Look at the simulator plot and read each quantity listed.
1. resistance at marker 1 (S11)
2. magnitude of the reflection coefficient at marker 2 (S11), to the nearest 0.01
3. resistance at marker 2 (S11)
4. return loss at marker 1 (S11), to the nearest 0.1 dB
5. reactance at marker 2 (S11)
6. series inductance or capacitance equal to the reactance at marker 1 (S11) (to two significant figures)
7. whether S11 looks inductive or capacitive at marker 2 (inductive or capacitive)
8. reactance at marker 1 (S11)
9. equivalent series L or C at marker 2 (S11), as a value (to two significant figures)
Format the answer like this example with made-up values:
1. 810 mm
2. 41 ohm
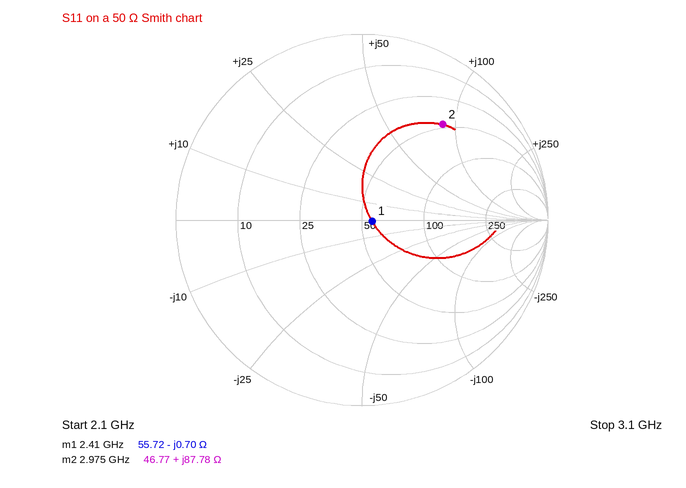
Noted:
1. 55.72 Ω
2. 0.67
3. 46.77 Ω
4. 25.3 dB
5. +87.78 Ω
6. 94 pF
7. inductive
8. -0.70 Ω
9. 4.7 nH
